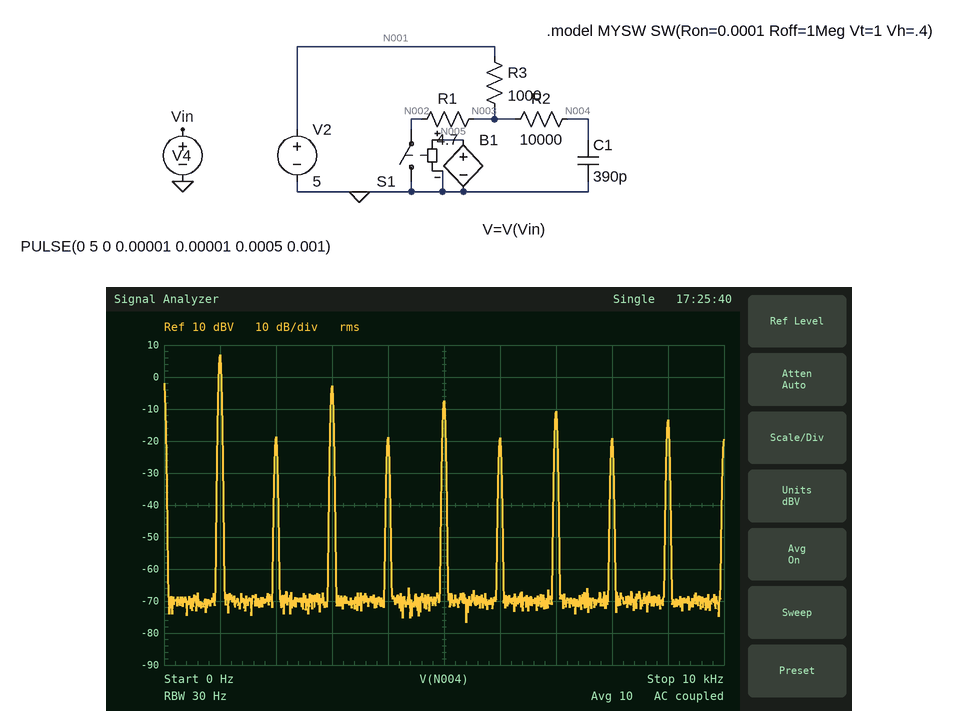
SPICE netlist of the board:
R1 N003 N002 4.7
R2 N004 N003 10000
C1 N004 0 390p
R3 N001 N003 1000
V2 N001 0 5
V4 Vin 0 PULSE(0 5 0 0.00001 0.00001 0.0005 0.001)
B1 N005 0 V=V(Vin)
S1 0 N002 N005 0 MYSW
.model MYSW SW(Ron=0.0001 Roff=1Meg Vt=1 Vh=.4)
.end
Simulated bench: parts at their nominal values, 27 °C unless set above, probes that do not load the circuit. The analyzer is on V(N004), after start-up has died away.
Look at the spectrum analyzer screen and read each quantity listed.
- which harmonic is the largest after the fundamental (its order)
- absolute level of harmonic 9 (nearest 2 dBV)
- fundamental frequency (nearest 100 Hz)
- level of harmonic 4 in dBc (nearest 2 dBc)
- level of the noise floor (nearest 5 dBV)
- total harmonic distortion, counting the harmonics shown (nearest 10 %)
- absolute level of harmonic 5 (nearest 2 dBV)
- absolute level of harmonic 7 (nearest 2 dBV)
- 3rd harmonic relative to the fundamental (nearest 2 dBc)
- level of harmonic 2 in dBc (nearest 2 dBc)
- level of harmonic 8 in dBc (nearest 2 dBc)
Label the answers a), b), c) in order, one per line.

a) 3
b) -14 dBV
c) 1.0 kHz
d) -26 dBc
e) -70 dBV
f) 40 %
g) -8 dBV
h) -10 dBV
i) -10 dBc
j) -26 dBc
k) -26 dBc
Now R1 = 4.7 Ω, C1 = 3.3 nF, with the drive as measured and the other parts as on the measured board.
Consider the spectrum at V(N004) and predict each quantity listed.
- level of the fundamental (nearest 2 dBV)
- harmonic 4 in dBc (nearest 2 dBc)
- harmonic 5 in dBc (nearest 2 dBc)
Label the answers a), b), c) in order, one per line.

a) 6 dBV
b) -28 dBc
c) -18 dBc
